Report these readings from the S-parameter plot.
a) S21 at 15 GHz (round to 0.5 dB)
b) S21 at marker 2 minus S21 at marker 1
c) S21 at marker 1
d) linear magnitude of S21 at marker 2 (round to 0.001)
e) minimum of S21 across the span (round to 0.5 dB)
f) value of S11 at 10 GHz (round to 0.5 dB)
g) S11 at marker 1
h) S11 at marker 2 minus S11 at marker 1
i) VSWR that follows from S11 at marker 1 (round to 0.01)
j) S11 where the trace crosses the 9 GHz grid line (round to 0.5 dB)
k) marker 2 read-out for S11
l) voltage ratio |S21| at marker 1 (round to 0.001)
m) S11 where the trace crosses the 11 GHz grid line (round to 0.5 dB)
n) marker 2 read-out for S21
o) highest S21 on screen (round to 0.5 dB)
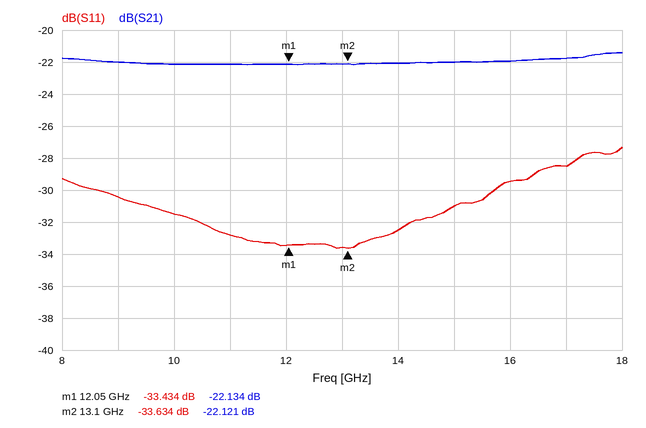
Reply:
-22.0 dB
0.013 dB
-22.134 dB
0.078
-22.0 dB
-31.5 dB
-33.434 dB
-0.200 dB
1.04
-30.5 dB
-33.634 dB
0.078
-33.0 dB
-22.121 dB
-21.5 dB
